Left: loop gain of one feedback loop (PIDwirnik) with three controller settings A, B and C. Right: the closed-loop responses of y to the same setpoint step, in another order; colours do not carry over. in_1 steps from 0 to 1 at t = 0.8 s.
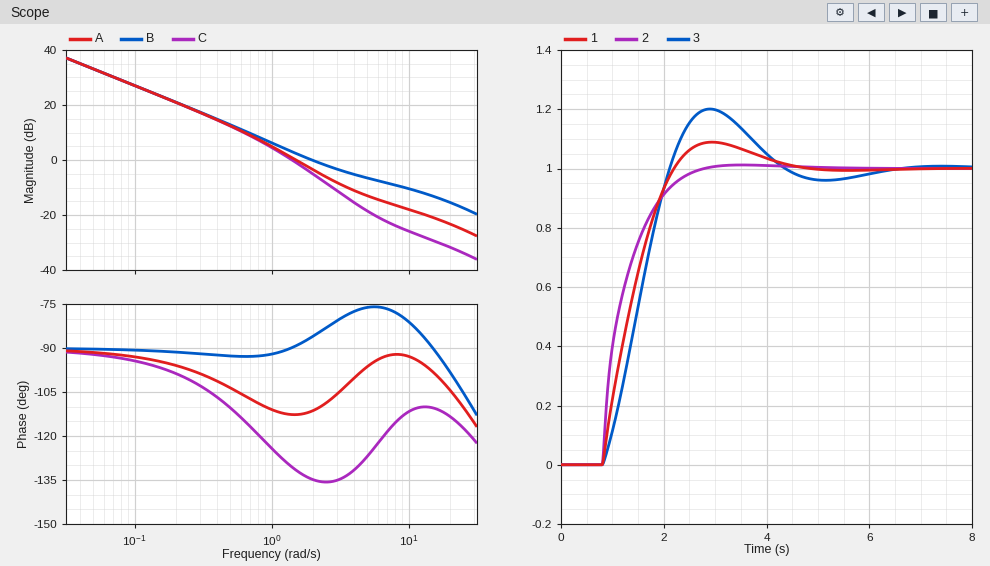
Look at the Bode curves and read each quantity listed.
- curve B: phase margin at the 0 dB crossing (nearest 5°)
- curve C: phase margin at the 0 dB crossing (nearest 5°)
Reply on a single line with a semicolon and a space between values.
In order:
95°; 50°
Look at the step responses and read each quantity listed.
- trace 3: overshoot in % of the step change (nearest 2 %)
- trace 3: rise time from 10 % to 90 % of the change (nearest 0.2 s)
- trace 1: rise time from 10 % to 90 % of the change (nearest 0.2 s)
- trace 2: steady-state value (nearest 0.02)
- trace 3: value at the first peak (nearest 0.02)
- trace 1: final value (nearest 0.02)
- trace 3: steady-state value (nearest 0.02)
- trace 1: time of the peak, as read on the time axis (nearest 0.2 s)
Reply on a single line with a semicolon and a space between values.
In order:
20 %; 1.0 s; 1.0 s; 1.00; 1.20; 1.00; 1.00; 3.0 s
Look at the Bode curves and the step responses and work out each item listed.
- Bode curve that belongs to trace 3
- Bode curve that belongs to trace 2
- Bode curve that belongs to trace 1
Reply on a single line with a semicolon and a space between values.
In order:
C; B; A
